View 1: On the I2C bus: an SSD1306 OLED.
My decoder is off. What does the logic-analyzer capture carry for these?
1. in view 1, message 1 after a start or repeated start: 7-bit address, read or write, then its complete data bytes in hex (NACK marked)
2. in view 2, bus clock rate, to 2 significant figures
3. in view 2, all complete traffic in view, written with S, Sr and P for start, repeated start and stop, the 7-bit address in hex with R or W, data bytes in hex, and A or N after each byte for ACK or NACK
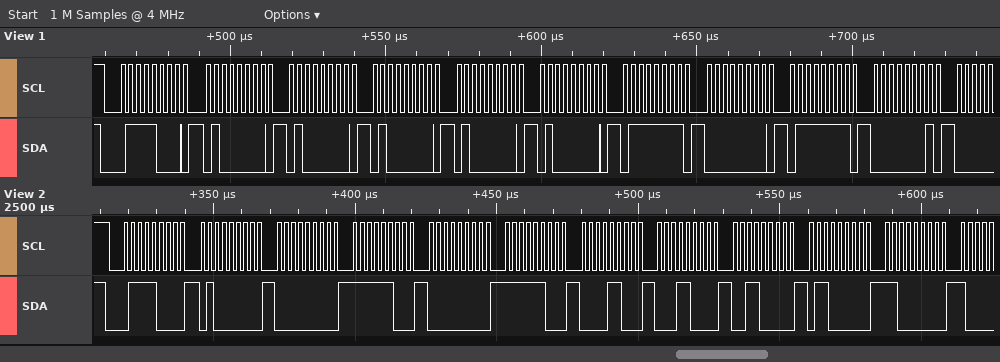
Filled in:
0x3C write: 40 40 40 40 40 7F 00 7F 01
400 kHz
S 3CW A 40 A 00 A FC A 00 A FC A 0C A 18 A 30 A 60 A C0 A
